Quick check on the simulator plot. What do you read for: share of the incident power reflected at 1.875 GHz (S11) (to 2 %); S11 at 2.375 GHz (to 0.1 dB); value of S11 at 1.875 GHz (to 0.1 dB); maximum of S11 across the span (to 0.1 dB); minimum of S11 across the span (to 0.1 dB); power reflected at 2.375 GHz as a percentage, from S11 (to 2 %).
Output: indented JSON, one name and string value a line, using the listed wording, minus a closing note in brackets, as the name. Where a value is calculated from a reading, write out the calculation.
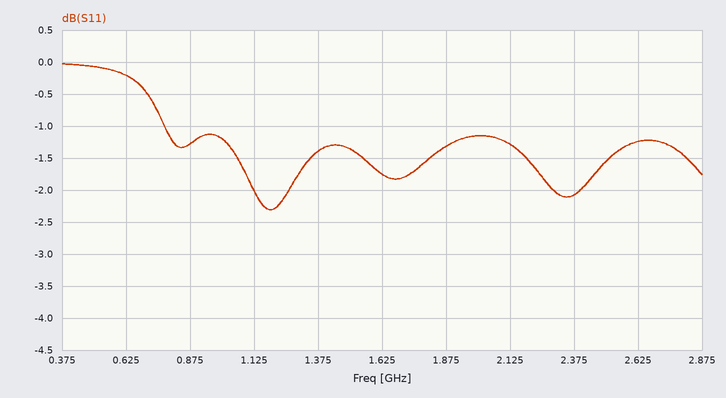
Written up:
{
  "share of the incident power reflected at 1.875 GHz (S11)": "10^(-1.3/10) ≈ 74 %",
  "S11 at 2.375 GHz": "-2.1 dB",
  "value of S11 at 1.875 GHz": "-1.3 dB",
  "maximum of S11 across the span": "0.0 dB",
  "minimum of S11 across the span": "-2.3 dB",
  "power reflected at 2.375 GHz as a percentage, from S11": "10^(-2.1/10) ≈ 62 %"
}
